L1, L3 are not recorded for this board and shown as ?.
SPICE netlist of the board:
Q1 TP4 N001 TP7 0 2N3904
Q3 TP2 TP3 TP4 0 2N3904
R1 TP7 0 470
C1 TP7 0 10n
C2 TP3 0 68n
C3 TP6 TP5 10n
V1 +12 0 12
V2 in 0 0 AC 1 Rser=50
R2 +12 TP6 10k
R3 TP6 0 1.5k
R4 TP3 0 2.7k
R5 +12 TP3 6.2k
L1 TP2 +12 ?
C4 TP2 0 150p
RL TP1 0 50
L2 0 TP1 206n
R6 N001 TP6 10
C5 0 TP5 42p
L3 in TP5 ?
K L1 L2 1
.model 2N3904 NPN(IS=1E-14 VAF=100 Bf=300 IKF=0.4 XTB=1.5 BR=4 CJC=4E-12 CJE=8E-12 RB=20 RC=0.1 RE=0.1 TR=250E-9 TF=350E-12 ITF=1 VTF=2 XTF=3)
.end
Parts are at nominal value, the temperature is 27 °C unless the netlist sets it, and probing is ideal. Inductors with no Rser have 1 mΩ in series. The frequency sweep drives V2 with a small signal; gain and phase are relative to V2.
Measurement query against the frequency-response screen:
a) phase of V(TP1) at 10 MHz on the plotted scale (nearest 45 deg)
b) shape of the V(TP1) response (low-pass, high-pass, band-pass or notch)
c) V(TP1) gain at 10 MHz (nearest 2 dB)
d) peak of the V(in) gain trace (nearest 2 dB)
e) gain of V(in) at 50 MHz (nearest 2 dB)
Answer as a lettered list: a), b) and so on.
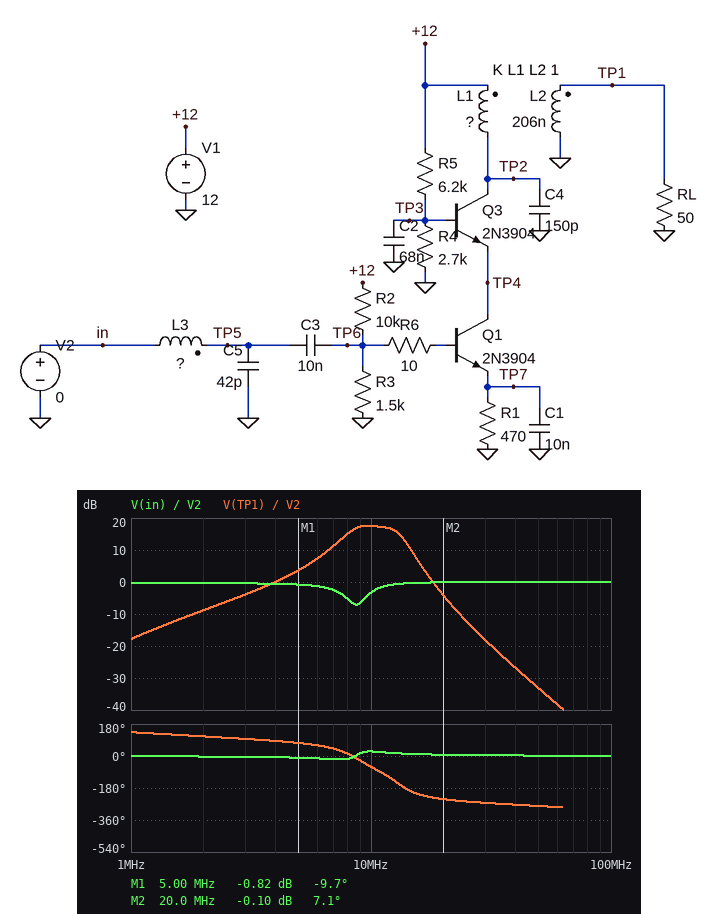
a) -45 deg
b) band-pass
c) 18 dB
d) 0 dB
e) 0 dB
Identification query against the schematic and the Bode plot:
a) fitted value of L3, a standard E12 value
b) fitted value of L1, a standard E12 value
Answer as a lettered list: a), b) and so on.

a) 3.9 µH
b) 1 µH
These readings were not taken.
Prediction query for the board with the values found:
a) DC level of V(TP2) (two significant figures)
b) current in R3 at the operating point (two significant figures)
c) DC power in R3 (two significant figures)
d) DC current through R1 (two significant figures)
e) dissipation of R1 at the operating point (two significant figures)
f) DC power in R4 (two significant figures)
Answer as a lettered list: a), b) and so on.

a) 12 V
b) 1.0 mA
c) 1.6 mW
d) 1.9 mA
e) 1.7 mW
f) 4.9 mW
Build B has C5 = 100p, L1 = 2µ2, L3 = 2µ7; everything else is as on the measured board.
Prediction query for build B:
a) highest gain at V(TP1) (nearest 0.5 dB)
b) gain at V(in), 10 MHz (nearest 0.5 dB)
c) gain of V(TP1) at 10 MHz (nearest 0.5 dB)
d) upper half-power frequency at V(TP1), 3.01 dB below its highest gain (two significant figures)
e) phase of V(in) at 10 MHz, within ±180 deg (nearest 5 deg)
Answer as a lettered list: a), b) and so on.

a) 27.0 dB
b) -3.0 dB
c) 19.5 dB
d) 9.3 MHz
e) 35 deg
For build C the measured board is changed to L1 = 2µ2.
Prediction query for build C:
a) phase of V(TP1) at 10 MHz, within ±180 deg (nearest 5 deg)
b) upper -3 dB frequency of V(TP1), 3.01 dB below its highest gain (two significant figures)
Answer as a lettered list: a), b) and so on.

a) -170 deg
b) 9.5 MHz
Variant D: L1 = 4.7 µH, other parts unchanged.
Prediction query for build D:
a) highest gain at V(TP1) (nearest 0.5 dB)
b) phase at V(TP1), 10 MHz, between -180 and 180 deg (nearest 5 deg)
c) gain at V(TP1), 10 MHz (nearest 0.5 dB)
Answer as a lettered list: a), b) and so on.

a) 28.5 dB
b) 160 deg
c) 12.5 dB
